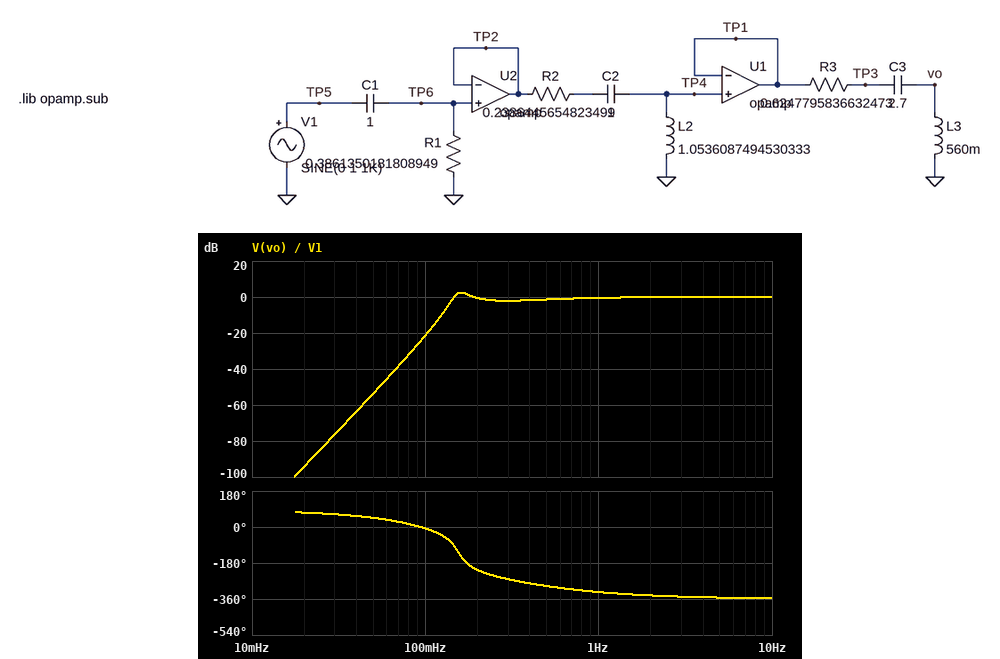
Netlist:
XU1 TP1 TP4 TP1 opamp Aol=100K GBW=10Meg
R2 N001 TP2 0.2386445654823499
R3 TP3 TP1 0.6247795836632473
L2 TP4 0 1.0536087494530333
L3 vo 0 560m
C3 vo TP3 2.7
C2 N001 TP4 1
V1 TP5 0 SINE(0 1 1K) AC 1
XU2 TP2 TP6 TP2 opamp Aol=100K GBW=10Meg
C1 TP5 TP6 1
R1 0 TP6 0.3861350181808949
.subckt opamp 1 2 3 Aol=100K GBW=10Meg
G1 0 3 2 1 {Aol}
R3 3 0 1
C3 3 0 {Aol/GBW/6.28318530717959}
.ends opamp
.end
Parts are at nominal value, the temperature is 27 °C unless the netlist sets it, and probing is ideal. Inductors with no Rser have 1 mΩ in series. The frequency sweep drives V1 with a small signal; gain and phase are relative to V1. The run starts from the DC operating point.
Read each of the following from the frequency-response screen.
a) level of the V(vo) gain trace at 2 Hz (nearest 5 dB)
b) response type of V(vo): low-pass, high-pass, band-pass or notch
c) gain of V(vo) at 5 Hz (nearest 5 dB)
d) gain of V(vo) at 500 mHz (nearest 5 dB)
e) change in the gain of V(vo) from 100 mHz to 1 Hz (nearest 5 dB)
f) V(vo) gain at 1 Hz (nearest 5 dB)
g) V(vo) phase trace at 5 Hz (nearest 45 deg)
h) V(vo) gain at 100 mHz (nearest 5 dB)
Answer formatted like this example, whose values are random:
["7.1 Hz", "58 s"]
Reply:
["0 dB", "high-pass", "0 dB", "0 dB", "20 dB", "0 dB", "-360 deg", "-20 dB"]
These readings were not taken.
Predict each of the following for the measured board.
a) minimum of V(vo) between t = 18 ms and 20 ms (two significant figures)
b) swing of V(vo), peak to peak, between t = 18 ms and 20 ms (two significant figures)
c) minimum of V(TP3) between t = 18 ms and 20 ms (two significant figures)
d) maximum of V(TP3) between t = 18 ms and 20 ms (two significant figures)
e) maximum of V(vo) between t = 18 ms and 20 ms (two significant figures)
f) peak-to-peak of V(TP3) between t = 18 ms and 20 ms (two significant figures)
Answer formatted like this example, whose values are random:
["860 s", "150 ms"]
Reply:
["-1.0 V", "2.0 V", "-1.0 V", "1.0 V", "1.0 V", "2.0 V"]
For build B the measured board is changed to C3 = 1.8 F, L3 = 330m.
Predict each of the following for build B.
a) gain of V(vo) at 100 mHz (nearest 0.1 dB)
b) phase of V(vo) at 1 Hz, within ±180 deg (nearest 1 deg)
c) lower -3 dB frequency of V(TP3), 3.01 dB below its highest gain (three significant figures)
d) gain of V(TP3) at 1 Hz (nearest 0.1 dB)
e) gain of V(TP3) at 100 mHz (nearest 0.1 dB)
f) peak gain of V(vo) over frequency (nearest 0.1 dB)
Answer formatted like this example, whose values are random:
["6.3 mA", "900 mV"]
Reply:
["-28.7 dB", "42 deg", "521 mHz", "-0.9 dB", "-18.5 dB", "0 dB"]
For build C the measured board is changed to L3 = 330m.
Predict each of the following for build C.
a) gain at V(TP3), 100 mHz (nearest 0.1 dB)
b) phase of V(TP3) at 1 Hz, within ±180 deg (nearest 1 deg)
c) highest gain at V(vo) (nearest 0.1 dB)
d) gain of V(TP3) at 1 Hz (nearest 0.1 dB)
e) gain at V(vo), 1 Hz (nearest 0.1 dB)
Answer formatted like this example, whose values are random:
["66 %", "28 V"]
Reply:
["-21.4 dB", "42 deg", "0 dB", "-0.9 dB", "-0.6 dB"]
